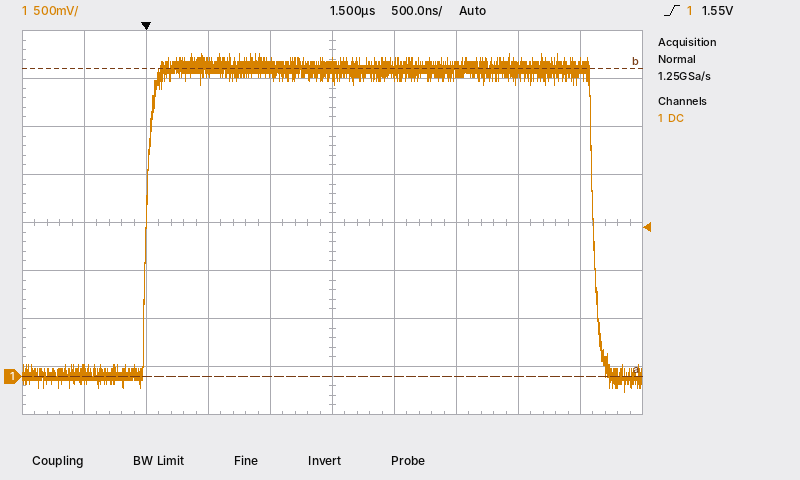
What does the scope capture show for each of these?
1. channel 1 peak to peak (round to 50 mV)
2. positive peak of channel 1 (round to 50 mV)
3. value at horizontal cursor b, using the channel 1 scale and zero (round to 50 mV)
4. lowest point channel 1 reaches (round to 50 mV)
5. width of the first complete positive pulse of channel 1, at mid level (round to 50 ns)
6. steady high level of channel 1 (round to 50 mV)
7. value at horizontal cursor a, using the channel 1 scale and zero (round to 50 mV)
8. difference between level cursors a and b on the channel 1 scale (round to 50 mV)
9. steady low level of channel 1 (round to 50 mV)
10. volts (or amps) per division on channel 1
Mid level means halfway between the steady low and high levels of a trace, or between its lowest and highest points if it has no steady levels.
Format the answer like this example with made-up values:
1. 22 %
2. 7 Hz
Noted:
1. 3.50 V
2. 3.35 V
3. 3.20 V
4. -150 mV
5. 3.60 µs
6. 3.20 V
7. 0 mV
8. 3.20 V
9. 0 mV
10. 500 mV
